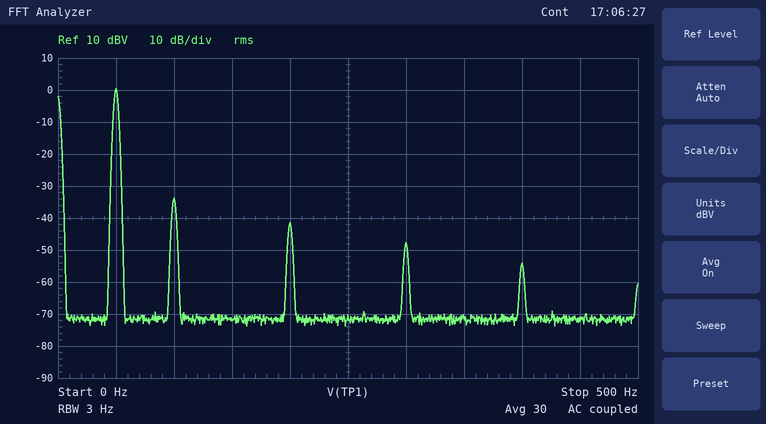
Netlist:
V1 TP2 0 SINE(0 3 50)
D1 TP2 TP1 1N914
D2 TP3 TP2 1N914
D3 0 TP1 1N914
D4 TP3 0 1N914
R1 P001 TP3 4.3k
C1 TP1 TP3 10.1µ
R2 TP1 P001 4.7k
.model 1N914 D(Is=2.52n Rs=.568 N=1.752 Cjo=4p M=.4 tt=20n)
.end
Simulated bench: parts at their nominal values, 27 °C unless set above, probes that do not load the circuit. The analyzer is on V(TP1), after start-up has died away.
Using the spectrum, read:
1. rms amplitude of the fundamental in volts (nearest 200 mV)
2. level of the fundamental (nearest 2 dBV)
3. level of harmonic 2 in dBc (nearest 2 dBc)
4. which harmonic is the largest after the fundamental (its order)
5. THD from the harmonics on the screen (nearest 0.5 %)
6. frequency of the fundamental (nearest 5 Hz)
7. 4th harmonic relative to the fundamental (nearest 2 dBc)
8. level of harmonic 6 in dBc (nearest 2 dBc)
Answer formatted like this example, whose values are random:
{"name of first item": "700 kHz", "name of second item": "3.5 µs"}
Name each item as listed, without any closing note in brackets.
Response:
{"rms amplitude of the fundamental in volts": "1.0 V", "level of the fundamental": "0 dBV", "level of harmonic 2 in dBc": "-34 dBc", "which harmonic is the largest after the fundamental": "2", "THD from the harmonics on the screen": "2.0 %", "frequency of the fundamental": "50 Hz", "4th harmonic relative to the fundamental": "-42 dBc", "level of harmonic 6 in dBc": "-48 dBc"}
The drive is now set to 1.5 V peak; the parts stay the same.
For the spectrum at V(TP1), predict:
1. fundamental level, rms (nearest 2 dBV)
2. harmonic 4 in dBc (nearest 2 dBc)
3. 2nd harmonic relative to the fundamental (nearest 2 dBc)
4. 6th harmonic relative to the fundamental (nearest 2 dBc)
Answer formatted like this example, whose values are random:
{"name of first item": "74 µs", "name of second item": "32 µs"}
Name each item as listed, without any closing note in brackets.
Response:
{"fundamental level, rms": "-6 dBV", "harmonic 4 in dBc": "-50 dBc", "2nd harmonic relative to the fundamental": "-40 dBc", "6th harmonic relative to the fundamental": "-58 dBc"}
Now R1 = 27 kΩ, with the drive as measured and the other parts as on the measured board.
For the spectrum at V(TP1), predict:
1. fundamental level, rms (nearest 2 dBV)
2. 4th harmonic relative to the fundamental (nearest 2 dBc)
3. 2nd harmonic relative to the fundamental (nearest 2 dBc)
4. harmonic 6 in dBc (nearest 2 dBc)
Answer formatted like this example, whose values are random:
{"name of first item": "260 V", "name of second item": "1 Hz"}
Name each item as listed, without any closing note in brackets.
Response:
{"fundamental level, rms": "0 dBV", "4th harmonic relative to the fundamental": "-52 dBc", "2nd harmonic relative to the fundamental": "-44 dBc", "harmonic 6 in dBc": "-58 dBc"}
